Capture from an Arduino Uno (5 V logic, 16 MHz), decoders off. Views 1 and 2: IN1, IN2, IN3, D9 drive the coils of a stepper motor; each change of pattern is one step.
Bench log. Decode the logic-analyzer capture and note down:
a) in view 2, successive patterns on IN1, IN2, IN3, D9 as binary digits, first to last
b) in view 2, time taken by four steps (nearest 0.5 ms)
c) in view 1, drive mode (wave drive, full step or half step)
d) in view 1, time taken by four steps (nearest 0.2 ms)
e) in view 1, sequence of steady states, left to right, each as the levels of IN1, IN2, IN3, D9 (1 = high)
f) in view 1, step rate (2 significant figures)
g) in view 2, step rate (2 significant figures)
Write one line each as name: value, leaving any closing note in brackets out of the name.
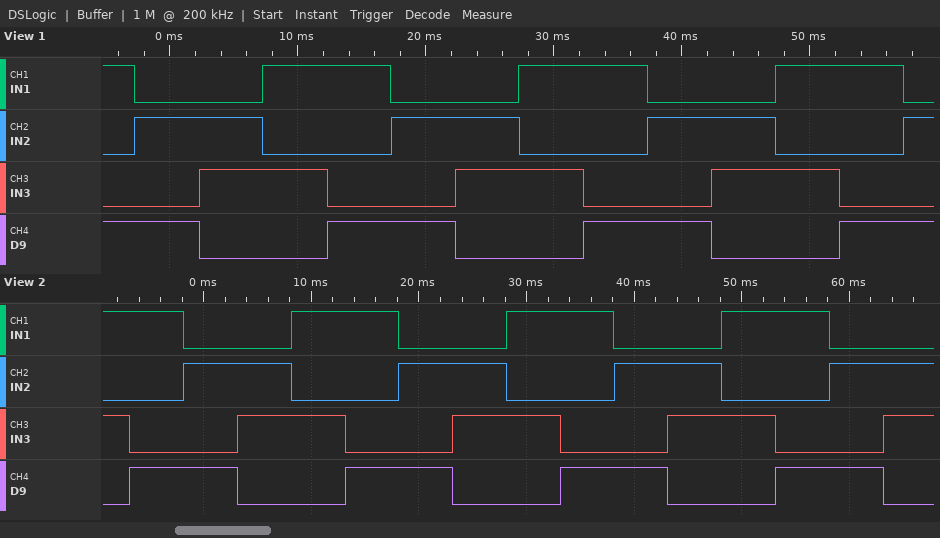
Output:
in view 2, successive patterns on IN1, IN2, IN3, D9 as binary digits, first to last: 1010 1001 0101 0110 1010 1001 0101 0110 1010 1001 0101 0110 1010 1001 0101 0110
in view 2, time taken by four steps: 20.0 ms
in view 1, drive mode: full step
in view 1, time taken by four steps: 20.0 ms
in view 1, sequence of steady states, left to right, each as the levels of IN1, IN2, IN3, D9: 1001 0101 0110 1010 1001 0101 0110 1010 1001 0101 0110 1010 1001 0101
in view 1, step rate: 200 steps/s
in view 2, step rate: 200 steps/s
